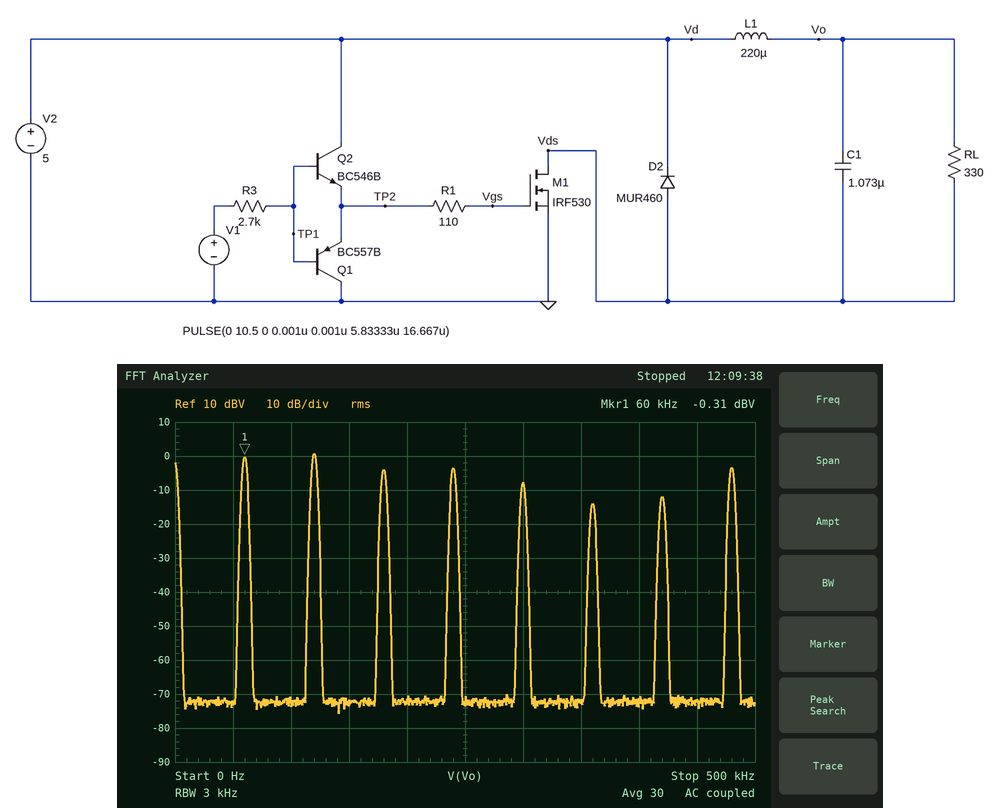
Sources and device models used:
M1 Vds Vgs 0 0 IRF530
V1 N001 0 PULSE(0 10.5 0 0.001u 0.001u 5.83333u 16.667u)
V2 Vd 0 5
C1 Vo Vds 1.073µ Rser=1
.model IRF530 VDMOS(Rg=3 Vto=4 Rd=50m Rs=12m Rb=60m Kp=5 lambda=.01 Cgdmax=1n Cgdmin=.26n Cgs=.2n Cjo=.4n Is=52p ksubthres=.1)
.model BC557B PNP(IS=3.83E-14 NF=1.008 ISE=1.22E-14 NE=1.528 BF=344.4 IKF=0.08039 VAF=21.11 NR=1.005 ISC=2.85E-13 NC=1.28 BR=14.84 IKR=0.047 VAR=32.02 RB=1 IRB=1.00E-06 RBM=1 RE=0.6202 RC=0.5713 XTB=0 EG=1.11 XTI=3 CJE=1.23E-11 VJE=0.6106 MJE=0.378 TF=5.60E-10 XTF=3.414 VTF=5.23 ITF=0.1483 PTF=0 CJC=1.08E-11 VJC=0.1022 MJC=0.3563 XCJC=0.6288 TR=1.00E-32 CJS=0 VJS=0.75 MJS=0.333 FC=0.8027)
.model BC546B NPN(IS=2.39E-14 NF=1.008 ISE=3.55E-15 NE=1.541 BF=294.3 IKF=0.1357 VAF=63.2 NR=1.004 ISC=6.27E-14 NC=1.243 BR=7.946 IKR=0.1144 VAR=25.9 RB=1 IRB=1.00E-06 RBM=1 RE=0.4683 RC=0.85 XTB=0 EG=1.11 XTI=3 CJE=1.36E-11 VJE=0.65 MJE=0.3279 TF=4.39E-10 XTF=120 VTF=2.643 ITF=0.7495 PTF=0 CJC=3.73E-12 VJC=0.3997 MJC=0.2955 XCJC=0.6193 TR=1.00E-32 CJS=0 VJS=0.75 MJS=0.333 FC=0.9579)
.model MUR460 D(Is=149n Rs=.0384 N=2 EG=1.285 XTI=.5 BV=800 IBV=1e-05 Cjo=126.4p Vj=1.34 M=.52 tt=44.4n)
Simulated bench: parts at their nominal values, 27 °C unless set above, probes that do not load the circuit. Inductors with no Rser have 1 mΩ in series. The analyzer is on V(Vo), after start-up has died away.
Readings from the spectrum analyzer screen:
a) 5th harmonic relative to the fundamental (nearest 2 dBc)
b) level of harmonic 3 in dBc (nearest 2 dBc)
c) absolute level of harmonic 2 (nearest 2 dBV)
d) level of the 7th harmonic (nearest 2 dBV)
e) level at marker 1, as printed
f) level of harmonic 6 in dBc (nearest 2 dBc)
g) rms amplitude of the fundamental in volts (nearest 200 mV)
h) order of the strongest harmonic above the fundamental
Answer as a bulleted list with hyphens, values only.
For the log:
- -8 dBc
- -4 dBc
- 0 dBV
- -12 dBV
- -0.31 dBV
- -14 dBc
- 1.0 V
- 2
